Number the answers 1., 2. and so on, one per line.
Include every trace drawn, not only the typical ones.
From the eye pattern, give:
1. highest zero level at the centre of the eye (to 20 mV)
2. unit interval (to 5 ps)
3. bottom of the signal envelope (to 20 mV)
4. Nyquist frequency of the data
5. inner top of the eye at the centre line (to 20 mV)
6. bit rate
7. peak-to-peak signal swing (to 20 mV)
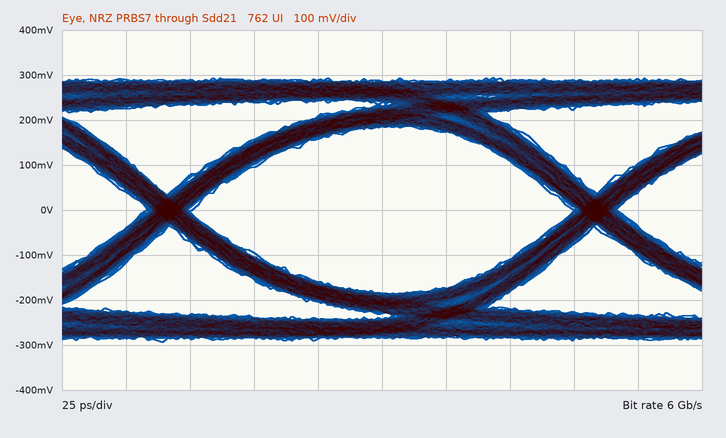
1. -180 mV
2. 165 ps
3. -300 mV
4. 3 GHz
5. 180 mV
6. 6 Gb/s
7. 580 mV
